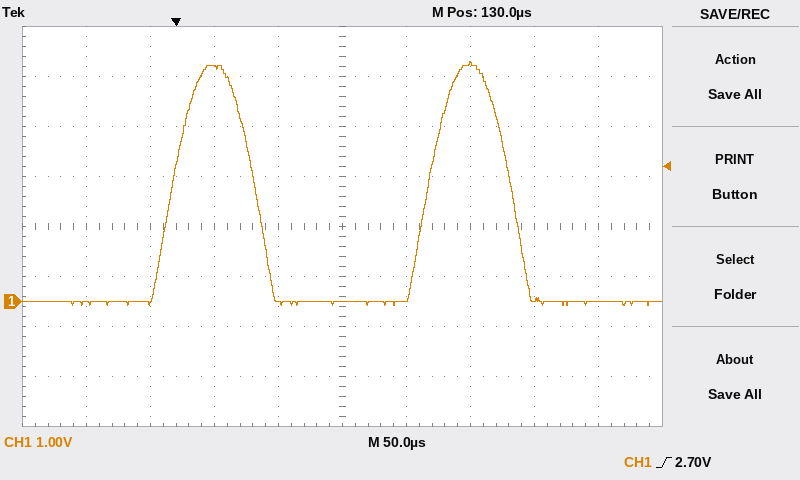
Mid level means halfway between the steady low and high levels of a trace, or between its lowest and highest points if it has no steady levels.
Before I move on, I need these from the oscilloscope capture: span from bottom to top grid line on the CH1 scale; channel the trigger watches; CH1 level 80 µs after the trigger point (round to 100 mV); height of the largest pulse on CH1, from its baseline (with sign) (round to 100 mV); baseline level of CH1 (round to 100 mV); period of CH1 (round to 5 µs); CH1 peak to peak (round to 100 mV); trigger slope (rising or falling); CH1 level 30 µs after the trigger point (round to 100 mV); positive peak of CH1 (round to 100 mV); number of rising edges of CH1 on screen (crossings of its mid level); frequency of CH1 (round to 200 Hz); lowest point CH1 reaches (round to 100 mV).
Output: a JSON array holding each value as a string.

["8 V", "CH1", "0.0 V", "+4.8 V", "0.0 V", "200 µs", "4.9 V", "rising", "4.7 V", "4.8 V", "2", "5.0 kHz", "-100 mV"]
